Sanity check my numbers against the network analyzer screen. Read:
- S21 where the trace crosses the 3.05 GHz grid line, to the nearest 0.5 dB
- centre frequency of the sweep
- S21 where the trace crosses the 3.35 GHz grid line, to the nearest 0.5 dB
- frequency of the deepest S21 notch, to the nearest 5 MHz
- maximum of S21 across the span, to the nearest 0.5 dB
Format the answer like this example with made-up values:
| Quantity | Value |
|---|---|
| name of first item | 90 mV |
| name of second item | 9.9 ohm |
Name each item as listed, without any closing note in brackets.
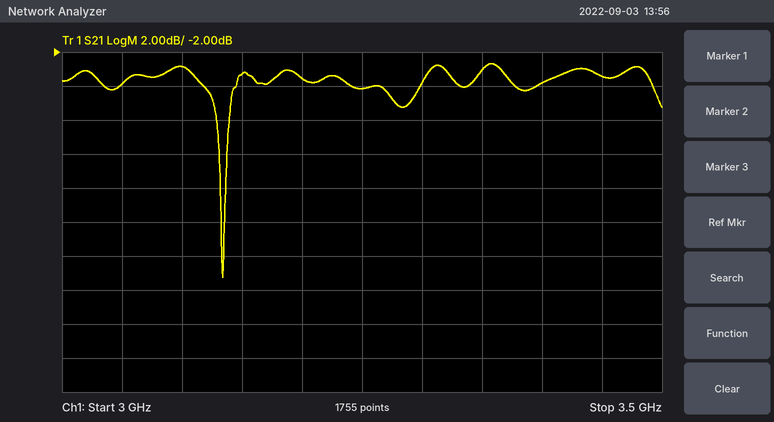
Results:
| Quantity | Value |
|---|---|
| S21 where the trace crosses the 3.05 GHz grid line, to the nearest 0.5 dB | -4.0 dB |
| centre frequency of the sweep | 3.25 GHz |
| S21 where the trace crosses the 3.35 GHz grid line, to the nearest 0.5 dB | -3.0 dB |
| frequency of the deepest S21 notch, to the nearest 5 MHz | 3.135 GHz |
| maximum of S21 across the span, to the nearest 0.5 dB | -2.5 dB |
